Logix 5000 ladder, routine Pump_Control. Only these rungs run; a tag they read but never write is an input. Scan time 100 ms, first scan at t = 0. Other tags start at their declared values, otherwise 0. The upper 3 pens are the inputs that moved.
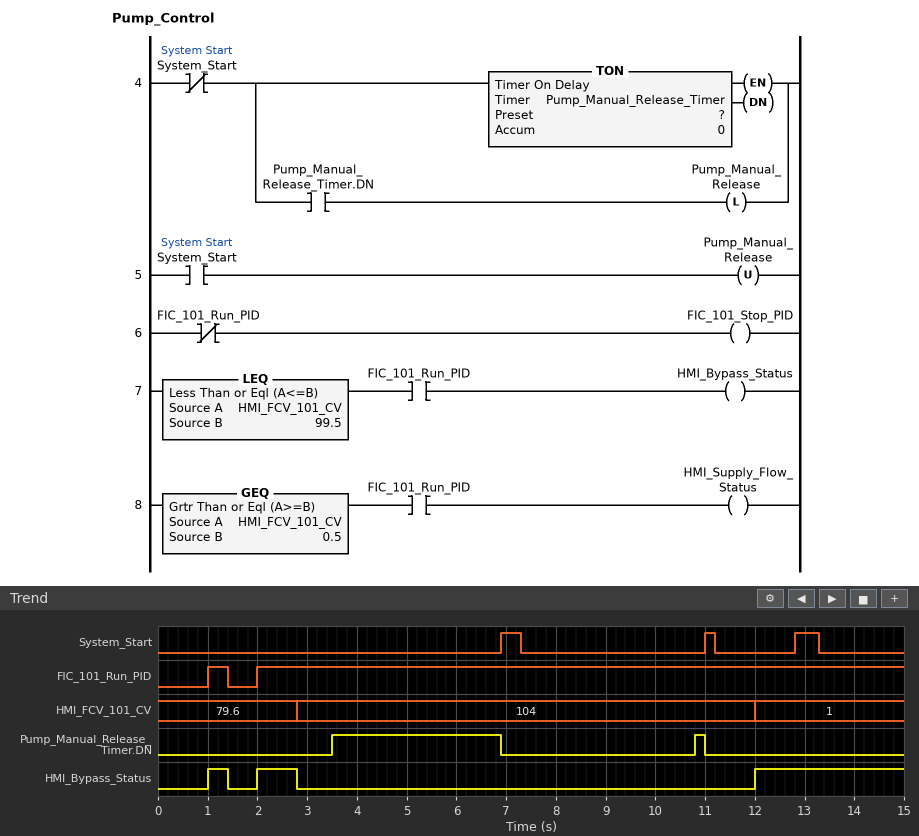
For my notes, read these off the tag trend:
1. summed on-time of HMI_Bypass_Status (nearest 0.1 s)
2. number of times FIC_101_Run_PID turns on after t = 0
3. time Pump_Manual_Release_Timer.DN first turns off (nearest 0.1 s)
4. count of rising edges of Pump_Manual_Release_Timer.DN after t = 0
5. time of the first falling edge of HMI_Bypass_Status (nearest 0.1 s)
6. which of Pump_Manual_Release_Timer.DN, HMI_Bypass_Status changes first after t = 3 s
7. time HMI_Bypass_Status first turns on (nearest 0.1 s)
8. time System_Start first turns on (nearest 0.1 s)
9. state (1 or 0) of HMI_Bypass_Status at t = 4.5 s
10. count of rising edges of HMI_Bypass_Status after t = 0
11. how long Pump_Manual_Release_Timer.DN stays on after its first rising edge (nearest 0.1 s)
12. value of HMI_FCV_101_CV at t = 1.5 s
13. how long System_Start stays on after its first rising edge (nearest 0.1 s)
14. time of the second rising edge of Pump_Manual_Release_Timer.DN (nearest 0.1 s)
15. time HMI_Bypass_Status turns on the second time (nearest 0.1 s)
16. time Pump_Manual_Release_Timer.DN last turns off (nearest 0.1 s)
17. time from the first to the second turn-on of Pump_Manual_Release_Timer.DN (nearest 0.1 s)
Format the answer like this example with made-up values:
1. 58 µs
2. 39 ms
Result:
1. 4.2 s
2. 2
3. 6.9 s
4. 2
5. 1.4 s
6. Pump_Manual_Release_Timer.DN
7. 1.0 s
8. 6.9 s
9. 0
10. 3
11. 3.4 s
12. 79.6
13. 0.4 s
14. 10.8 s
15. 2.0 s
16. 11.0 s
17. 7.3 s
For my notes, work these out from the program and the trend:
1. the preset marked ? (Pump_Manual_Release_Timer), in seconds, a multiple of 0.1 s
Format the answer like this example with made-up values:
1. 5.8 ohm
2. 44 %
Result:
1. 3.5 s
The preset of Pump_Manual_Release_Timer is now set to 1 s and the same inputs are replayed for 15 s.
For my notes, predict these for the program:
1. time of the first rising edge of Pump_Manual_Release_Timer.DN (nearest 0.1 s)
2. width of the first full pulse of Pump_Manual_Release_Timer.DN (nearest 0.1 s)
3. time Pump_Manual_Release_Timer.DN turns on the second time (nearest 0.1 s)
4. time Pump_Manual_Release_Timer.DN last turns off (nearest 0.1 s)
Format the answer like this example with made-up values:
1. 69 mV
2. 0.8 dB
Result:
1. 1.0 s
2. 5.9 s
3. 8.3 s
4. 12.8 s
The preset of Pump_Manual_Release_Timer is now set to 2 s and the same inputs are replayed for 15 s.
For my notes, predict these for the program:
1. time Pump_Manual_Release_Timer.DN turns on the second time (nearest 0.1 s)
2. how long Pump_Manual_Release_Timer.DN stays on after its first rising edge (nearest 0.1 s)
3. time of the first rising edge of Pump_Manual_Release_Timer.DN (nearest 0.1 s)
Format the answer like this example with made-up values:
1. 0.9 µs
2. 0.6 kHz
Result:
1. 9.3 s
2. 4.9 s
3. 2.0 s
